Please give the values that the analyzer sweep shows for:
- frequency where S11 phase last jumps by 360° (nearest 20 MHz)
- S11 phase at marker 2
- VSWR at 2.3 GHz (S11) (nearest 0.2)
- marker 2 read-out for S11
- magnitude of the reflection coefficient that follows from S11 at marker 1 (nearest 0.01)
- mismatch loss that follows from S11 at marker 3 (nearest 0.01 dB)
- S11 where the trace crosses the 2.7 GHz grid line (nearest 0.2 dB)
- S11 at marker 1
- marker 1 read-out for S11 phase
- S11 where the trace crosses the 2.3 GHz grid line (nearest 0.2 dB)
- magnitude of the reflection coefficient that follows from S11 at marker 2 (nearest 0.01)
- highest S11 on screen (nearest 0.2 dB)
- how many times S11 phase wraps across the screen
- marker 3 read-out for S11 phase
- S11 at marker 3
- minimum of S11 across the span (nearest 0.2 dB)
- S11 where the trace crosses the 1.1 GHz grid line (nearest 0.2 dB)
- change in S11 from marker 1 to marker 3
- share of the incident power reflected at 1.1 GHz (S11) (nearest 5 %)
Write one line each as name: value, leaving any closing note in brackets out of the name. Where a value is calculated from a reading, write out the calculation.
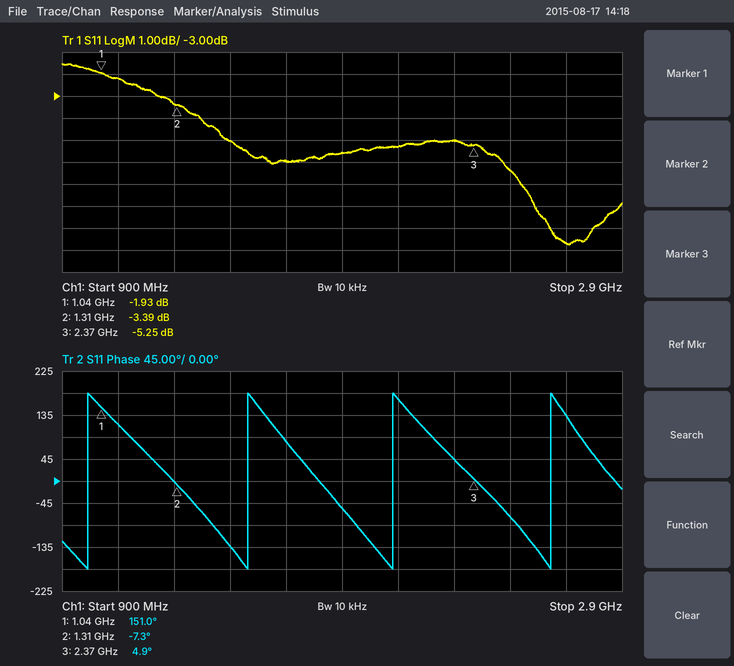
frequency where S11 phase last jumps by 360°: 2.64 GHz
S11 phase at marker 2: -7.3°
VSWR at 2.3 GHz (S11): |Γ| = 10^(-5/20) = 0.5623; VSWR = (1 + 0.5623)/(1 − 0.5623) ≈ 3.6
marker 2 read-out for S11: -3.39 dB
magnitude of the reflection coefficient that follows from S11 at marker 1: 10^(-1.93/20) ≈ 0.80
mismatch loss that follows from S11 at marker 3: −10 log10(1 − 10^(-5.25/10)) ≈ 1.54 dB
S11 where the trace crosses the 2.7 GHz grid line: -9.6 dB
S11 at marker 1: -1.93 dB
marker 1 read-out for S11 phase: 151.0°
S11 where the trace crosses the 2.3 GHz grid line: -5.0 dB
magnitude of the reflection coefficient that follows from S11 at marker 2: 10^(-3.39/20) ≈ 0.68
highest S11 on screen: -1.6 dB
how many times S11 phase wraps across the screen: 4
marker 3 read-out for S11 phase: 4.9°
S11 at marker 3: -5.25 dB
minimum of S11 across the span: -9.8 dB
S11 where the trace crosses the 1.1 GHz grid line: -2.2 dB
change in S11 from marker 1 to marker 3: -5.25 − (-1.93) = -3.32 dB
share of the incident power reflected at 1.1 GHz (S11): 10^(-2.2/10) ≈ 60 %
